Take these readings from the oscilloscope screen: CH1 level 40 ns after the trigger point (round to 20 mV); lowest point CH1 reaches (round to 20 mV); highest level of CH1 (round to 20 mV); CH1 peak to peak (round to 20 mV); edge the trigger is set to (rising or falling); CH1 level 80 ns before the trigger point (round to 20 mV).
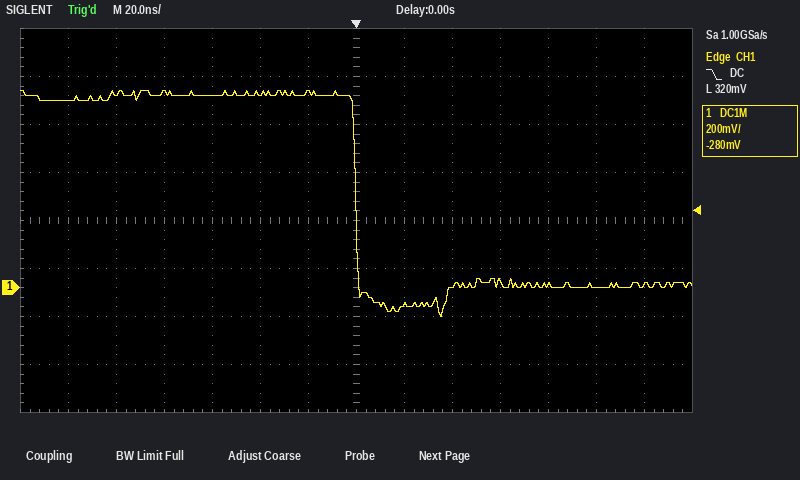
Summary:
0 mV
-120 mV
820 mV
940 mV
falling
820 mV
